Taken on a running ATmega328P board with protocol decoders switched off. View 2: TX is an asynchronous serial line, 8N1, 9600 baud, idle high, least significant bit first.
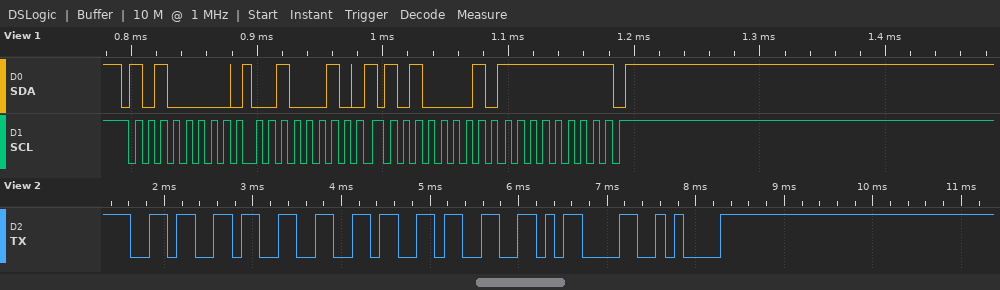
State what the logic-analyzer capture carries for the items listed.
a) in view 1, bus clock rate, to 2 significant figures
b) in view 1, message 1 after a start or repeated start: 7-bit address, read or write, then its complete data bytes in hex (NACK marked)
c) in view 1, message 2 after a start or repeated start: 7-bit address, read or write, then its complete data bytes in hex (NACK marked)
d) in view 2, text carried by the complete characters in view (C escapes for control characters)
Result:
100 kHz
0x50 write: 22
0x50 read: FF NACK
"6363\r\n"
